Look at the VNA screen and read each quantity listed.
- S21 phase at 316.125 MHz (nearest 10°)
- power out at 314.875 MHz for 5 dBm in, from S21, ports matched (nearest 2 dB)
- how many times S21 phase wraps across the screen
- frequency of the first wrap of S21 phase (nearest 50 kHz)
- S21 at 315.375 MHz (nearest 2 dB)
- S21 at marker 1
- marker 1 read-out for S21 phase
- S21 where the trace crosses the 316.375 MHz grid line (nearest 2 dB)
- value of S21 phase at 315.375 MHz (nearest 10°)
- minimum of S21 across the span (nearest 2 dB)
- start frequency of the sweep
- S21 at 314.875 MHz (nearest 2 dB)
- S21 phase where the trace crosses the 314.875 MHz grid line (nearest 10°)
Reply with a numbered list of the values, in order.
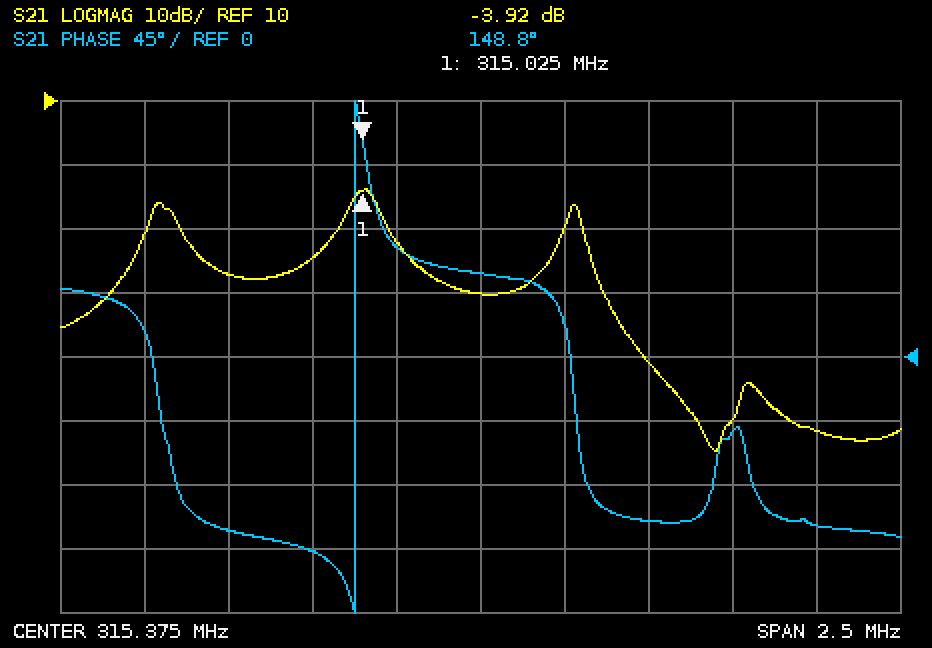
1. -50°
2. -10 dBm
3. 1
4. 315.00 MHz
5. -20 dB
6. -3.92 dB
7. 148.8°
8. -42 dB
9. 60°
10. -44 dB
11. 314.125 MHz
12. -14 dB
13. -140°
